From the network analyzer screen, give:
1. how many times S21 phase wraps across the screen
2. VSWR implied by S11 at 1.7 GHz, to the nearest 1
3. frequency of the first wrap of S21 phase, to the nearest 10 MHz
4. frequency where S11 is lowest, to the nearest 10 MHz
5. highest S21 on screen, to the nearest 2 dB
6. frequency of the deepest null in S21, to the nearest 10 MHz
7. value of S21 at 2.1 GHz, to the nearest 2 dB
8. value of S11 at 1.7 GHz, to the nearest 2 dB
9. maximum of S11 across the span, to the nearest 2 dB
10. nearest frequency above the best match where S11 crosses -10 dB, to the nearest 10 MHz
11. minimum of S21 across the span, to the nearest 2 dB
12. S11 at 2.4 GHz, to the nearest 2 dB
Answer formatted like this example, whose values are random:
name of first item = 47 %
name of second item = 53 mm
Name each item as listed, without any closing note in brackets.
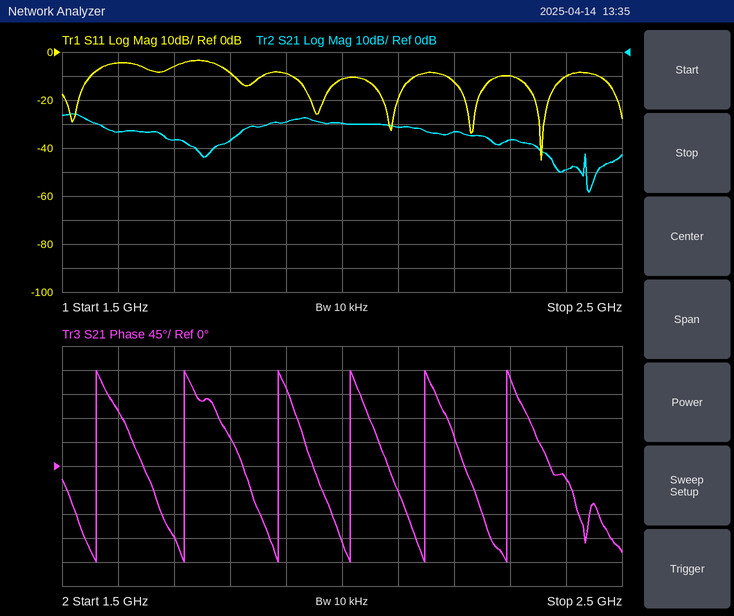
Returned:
how many times S21 phase wraps across the screen = 6
VSWR implied by S11 at 1.7 GHz, to the nearest 1 = 3
frequency of the first wrap of S21 phase, to the nearest 10 MHz = 1.56 GHz
frequency where S11 is lowest, to the nearest 10 MHz = 2.36 GHz
highest S21 on screen, to the nearest 2 dB = -26 dB
frequency of the deepest null in S21, to the nearest 10 MHz = 2.44 GHz
value of S21 at 2.1 GHz, to the nearest 2 dB = -32 dB
value of S11 at 1.7 GHz, to the nearest 2 dB = -6 dB
maximum of S11 across the span, to the nearest 2 dB = -4 dB
nearest frequency above the best match where S11 crosses -10 dB, to the nearest 10 MHz = 2.40 GHz
minimum of S21 across the span, to the nearest 2 dB = -58 dB
S11 at 2.4 GHz, to the nearest 2 dB = -10 dB
